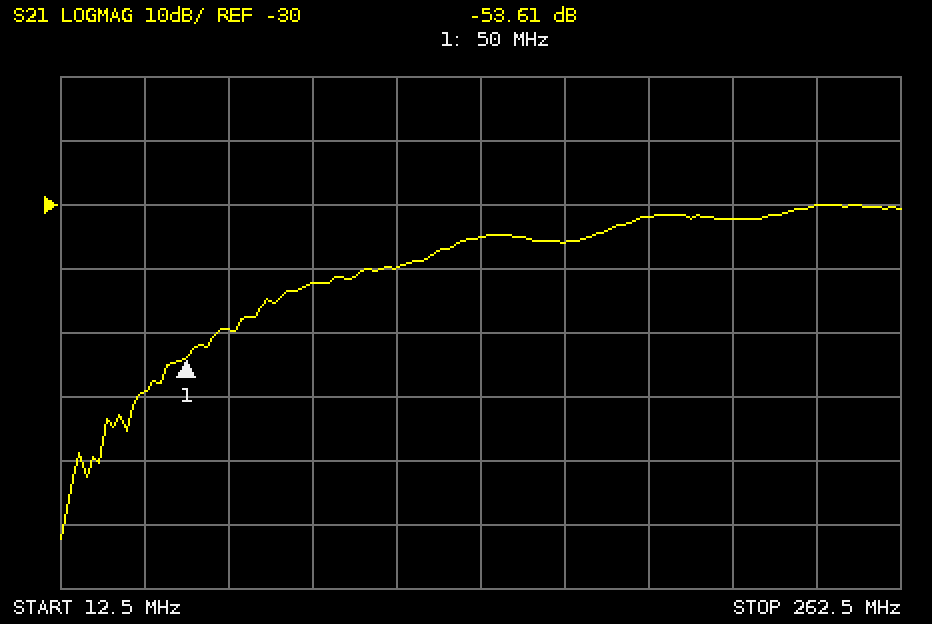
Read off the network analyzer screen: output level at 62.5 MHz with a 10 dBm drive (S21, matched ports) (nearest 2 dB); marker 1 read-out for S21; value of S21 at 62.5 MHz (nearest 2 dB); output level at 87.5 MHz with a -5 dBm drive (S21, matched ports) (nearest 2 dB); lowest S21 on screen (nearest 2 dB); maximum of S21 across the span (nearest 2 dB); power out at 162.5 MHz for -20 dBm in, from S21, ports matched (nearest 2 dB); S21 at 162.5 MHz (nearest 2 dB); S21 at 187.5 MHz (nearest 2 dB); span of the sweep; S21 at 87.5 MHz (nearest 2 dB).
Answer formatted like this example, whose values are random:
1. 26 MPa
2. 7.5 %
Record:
1. -40 dBm
2. -53.61 dB
3. -50 dB
4. -48 dBm
5. -82 dB
6. -30 dB
7. -56 dBm
8. -36 dB
9. -32 dB
10. 250 MHz
11. -42 dB
